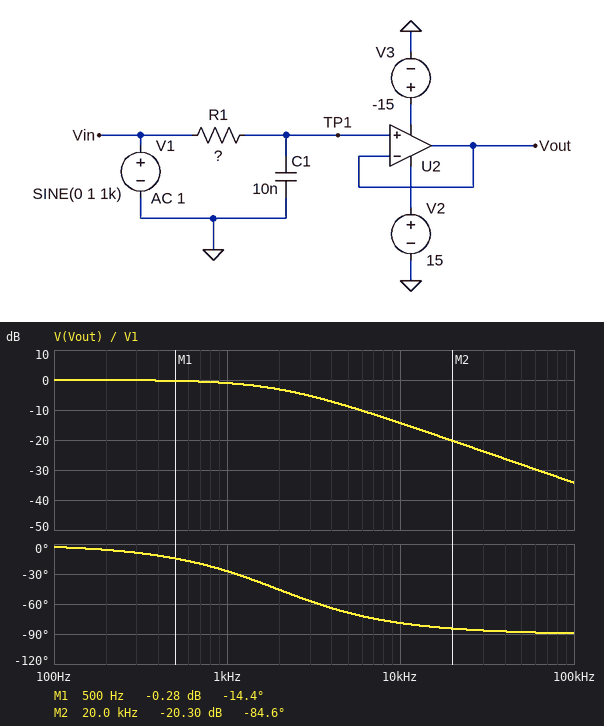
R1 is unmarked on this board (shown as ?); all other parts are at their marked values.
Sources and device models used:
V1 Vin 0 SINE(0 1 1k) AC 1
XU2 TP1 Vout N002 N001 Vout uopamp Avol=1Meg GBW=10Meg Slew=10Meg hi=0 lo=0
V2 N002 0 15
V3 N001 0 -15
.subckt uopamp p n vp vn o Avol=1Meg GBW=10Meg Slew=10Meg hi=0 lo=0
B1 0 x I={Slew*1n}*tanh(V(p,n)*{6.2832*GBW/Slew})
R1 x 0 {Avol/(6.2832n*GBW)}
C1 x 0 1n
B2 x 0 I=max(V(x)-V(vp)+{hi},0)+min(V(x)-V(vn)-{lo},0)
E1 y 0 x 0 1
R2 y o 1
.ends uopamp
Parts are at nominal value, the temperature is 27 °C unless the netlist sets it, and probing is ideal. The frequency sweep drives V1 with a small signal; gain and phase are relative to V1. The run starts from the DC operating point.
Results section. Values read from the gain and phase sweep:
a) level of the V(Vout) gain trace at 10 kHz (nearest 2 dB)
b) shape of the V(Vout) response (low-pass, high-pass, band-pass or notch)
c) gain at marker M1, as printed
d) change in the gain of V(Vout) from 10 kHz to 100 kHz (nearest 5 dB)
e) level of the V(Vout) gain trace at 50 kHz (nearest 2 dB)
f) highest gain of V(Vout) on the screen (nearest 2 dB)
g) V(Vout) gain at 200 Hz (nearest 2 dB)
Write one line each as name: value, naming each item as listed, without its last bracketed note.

level of the V(Vout) gain trace at 10 kHz: -14 dB
shape of the V(Vout) response: low-pass
gain at marker M1, as printed: -0.28 dB
change in the gain of V(Vout) from 10 kHz to 100 kHz: -20 dB
level of the V(Vout) gain trace at 50 kHz: -28 dB
highest gain of V(Vout) on the screen: 0 dB
V(Vout) gain at 200 Hz: 0 dB
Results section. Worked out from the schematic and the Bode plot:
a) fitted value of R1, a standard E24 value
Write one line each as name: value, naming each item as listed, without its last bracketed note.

fitted value of R1, a standard E24 value: 8.2 kΩ
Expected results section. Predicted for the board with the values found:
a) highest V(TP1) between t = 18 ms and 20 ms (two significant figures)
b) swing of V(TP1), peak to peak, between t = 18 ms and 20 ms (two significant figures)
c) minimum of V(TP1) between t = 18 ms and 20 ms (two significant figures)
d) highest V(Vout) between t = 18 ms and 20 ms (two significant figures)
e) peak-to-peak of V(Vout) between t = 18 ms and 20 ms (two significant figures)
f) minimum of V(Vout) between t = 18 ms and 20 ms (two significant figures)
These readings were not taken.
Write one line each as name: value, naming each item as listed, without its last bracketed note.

highest V(TP1) between t = 18 ms and 20 ms: 890 mV
swing of V(TP1), peak to peak, between t = 18 ms and 20 ms: 1.8 V
minimum of V(TP1) between t = 18 ms and 20 ms: -890 mV
highest V(Vout) between t = 18 ms and 20 ms: 890 mV
peak-to-peak of V(Vout) between t = 18 ms and 20 ms: 1.8 V
minimum of V(Vout) between t = 18 ms and 20 ms: -890 mV
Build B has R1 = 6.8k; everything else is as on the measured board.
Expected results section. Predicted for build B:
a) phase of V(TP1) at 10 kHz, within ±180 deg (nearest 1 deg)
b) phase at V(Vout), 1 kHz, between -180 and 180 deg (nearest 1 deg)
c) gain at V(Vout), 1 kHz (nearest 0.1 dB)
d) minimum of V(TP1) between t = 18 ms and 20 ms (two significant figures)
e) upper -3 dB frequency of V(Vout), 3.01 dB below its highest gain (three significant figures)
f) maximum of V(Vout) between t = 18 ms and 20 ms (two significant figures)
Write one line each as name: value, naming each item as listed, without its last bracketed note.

phase of V(TP1) at 10 kHz, within ±180 deg: -77 deg
phase at V(Vout), 1 kHz, between -180 and 180 deg: -23 deg
gain at V(Vout), 1 kHz: -0.7 dB
minimum of V(TP1) between t = 18 ms and 20 ms: -920 mV
upper -3 dB frequency of V(Vout), 3.01 dB below its highest gain: 2.34 kHz
maximum of V(Vout) between t = 18 ms and 20 ms: 920 mV
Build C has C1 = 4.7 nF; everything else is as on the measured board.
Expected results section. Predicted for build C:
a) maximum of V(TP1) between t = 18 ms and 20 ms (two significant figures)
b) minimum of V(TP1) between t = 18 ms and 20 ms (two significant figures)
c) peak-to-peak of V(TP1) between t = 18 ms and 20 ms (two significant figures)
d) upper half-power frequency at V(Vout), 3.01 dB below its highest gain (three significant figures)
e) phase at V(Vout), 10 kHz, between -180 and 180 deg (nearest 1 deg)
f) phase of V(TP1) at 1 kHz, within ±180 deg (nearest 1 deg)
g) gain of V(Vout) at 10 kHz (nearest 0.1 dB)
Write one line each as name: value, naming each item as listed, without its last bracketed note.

maximum of V(TP1) between t = 18 ms and 20 ms: 970 mV
minimum of V(TP1) between t = 18 ms and 20 ms: -970 mV
peak-to-peak of V(TP1) between t = 18 ms and 20 ms: 1.9 V
upper half-power frequency at V(Vout), 3.01 dB below its highest gain: 4.13 kHz
phase at V(Vout), 10 kHz, between -180 and 180 deg: -68 deg
phase of V(TP1) at 1 kHz, within ±180 deg: -14 deg
gain of V(Vout) at 10 kHz: -8.4 dB
